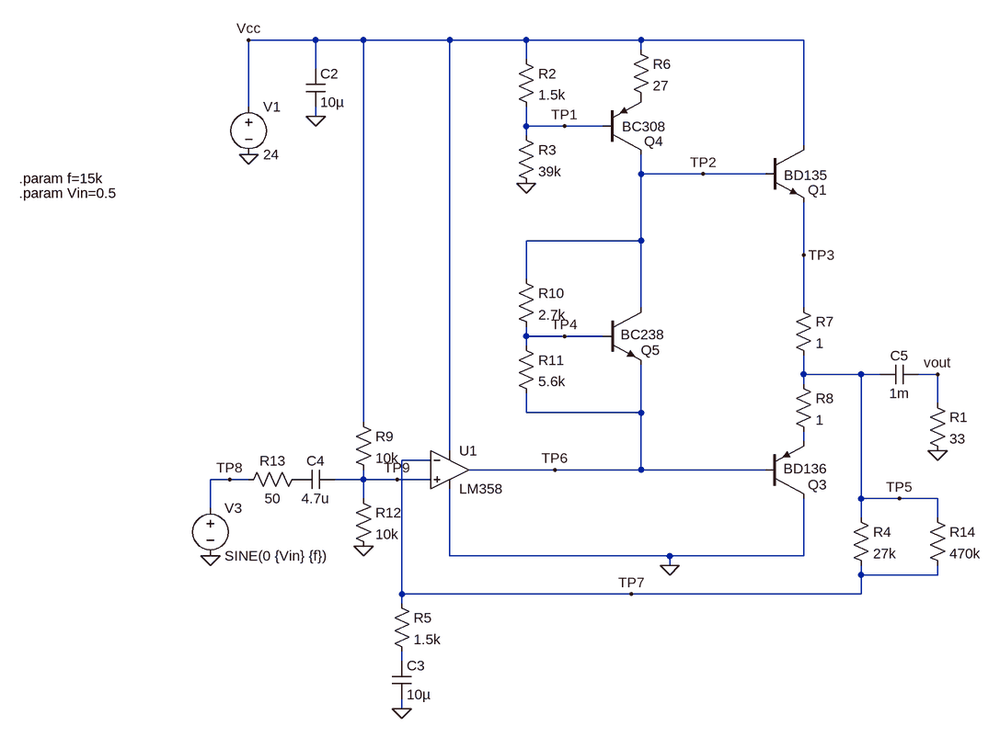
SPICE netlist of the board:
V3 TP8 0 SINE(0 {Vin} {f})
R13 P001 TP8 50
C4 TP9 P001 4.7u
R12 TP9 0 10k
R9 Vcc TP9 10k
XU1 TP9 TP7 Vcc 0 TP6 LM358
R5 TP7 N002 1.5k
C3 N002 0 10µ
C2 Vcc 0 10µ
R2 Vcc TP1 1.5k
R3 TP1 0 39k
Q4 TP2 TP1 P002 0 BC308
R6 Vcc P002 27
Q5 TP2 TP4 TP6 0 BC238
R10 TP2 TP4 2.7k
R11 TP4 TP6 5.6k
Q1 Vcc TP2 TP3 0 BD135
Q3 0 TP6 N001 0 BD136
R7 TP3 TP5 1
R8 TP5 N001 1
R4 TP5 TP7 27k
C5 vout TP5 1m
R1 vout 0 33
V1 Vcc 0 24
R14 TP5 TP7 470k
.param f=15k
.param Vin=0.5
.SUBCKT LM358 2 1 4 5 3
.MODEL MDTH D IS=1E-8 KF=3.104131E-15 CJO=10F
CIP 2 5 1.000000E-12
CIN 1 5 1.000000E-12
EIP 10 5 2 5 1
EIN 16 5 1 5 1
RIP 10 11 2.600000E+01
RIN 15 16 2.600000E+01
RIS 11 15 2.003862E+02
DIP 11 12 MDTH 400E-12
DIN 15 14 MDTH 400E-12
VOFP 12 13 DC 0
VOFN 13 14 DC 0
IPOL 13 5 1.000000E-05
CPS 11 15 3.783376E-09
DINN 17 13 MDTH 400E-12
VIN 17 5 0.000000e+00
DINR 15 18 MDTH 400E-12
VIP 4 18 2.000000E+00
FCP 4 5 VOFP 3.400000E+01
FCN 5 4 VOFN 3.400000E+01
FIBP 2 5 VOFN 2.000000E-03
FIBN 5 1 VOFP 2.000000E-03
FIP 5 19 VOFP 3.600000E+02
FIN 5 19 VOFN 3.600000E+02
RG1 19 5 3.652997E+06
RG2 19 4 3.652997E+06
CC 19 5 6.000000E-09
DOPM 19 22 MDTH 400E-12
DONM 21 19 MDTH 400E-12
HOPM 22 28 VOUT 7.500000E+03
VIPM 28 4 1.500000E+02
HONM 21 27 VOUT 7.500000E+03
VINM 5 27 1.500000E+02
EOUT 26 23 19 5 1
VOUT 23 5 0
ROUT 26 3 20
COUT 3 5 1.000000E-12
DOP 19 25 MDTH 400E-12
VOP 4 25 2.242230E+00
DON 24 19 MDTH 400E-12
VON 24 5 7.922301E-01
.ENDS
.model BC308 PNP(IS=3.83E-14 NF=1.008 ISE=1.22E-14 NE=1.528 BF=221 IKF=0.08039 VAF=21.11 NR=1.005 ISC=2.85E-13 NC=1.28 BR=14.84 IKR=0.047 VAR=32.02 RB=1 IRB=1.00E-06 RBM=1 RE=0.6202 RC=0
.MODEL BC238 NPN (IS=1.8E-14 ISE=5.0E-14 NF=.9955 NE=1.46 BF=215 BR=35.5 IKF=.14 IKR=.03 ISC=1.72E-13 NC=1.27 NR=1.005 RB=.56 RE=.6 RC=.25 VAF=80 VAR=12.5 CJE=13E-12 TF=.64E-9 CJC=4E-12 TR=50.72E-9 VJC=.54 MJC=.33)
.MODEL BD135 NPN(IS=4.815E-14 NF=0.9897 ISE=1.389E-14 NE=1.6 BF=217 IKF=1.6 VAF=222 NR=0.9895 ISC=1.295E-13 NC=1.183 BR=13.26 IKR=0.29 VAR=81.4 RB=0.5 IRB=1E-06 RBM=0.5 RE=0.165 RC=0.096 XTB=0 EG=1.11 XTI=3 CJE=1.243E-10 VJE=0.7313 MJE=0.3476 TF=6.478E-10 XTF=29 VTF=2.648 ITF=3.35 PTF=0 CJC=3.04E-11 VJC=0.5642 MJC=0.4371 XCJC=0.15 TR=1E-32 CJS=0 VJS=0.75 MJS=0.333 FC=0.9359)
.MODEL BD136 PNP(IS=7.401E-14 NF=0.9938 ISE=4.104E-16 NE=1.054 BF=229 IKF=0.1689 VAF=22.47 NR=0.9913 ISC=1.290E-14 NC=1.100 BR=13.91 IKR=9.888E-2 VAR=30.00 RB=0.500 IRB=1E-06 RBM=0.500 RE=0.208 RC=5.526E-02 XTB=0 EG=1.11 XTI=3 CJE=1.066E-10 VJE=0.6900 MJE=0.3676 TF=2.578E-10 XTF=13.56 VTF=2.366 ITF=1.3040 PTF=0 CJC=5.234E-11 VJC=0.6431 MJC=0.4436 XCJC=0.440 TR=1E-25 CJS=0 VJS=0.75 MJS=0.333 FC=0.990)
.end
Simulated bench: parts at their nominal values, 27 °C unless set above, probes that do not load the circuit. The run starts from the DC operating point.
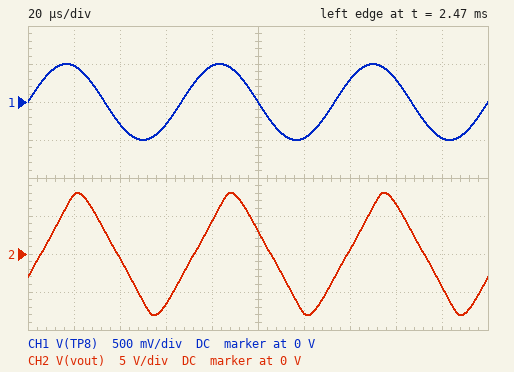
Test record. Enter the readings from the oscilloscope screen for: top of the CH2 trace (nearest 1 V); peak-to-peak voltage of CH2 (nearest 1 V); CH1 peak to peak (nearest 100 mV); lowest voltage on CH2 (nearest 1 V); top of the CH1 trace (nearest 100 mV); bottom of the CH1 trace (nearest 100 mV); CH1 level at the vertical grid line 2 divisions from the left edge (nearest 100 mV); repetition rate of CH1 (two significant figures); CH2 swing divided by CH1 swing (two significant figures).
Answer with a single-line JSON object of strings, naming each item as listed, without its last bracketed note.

{"top of the CH2 trace": "8 V", "peak-to-peak voltage of CH2": "16 V", "CH1 peak to peak": "1.0 V", "lowest voltage on CH2": "-8 V", "top of the CH1 trace": "500 mV", "bottom of the CH1 trace": "-500 mV", "CH1 level at the vertical grid line 2 divisions from the left edge": "-300 mV", "repetition rate of CH1": "15 kHz", "CH2 swing divided by CH1 swing": "16"}
